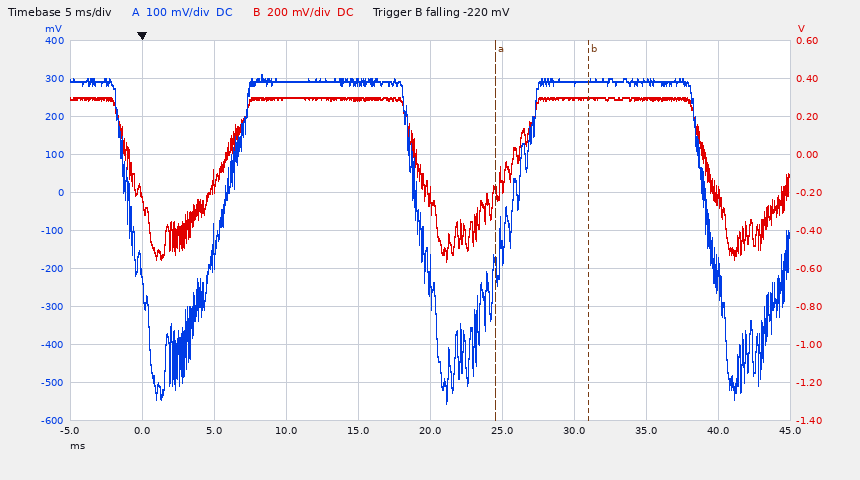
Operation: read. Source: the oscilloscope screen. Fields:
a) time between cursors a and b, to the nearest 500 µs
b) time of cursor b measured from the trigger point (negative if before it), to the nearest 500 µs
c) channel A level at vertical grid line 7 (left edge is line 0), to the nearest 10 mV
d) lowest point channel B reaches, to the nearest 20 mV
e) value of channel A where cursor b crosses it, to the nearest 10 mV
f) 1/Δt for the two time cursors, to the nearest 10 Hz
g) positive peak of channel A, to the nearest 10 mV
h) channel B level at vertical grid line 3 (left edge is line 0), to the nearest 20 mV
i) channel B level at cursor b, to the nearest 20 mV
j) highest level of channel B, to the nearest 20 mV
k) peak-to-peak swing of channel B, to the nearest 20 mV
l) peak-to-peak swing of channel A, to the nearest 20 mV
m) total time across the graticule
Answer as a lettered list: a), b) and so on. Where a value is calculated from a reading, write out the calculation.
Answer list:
a) 6.5 ms
b) +31.0 ms
c) 290 mV
d) -560 mV
e) 300 mV
f) 1 / 6.5 ms ≈ 150 Hz
g) 310 mV
h) 300 mV
i) 300 mV
j) 300 mV
k) 300 mV − (-560 mV) = 860 mV
l) 860 mV
m) 50 ms
